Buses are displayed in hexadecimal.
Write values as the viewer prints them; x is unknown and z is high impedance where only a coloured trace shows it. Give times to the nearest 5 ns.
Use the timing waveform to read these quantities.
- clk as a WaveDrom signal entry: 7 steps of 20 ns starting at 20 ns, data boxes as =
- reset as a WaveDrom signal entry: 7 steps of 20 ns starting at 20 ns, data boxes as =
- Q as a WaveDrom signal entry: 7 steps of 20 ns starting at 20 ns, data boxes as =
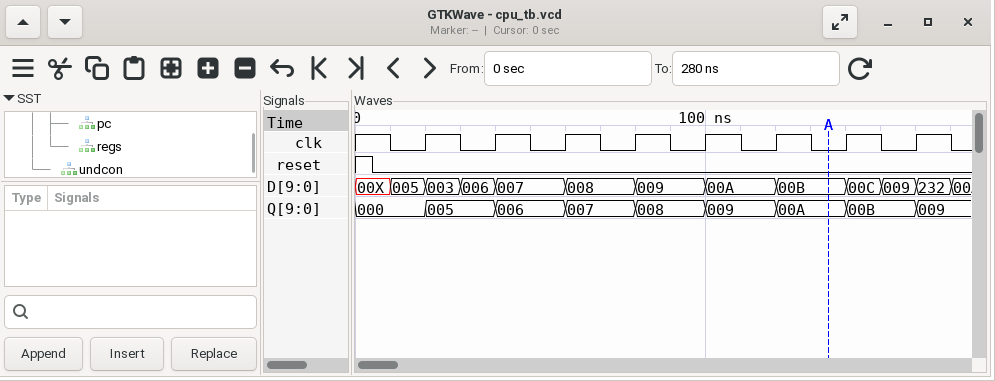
{name: 'clk', wave: 'p......'}
{name: 'reset', wave: '0......'}
{name: 'Q', wave: '=======', data: '005 006 007 008 009 00A 00B'}
